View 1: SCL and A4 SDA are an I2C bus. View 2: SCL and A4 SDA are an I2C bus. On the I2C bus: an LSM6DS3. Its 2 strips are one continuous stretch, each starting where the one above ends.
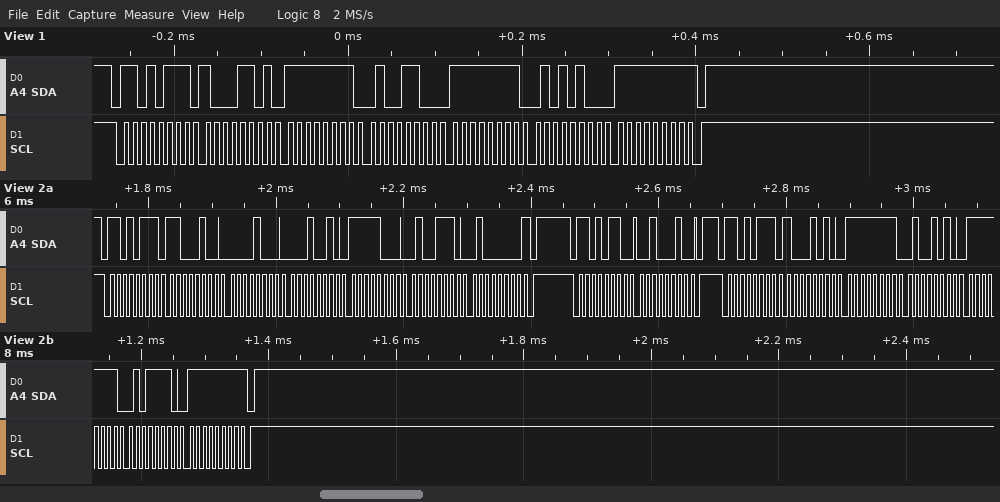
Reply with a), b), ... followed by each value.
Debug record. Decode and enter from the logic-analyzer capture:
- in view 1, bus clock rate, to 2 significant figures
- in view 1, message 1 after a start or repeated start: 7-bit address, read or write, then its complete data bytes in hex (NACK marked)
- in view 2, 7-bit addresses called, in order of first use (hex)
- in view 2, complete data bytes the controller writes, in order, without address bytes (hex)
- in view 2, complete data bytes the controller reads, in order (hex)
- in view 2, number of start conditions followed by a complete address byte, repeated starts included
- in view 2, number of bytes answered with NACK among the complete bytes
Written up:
a) 100 kHz
b) 0x6B read: 8D FF 4C FF 54 FF NACK
c) 0x6B
d) 22
e) C4 08 12 F8 4E 40 8A FF 4A FF 5E FF
f) 3
g) 2
